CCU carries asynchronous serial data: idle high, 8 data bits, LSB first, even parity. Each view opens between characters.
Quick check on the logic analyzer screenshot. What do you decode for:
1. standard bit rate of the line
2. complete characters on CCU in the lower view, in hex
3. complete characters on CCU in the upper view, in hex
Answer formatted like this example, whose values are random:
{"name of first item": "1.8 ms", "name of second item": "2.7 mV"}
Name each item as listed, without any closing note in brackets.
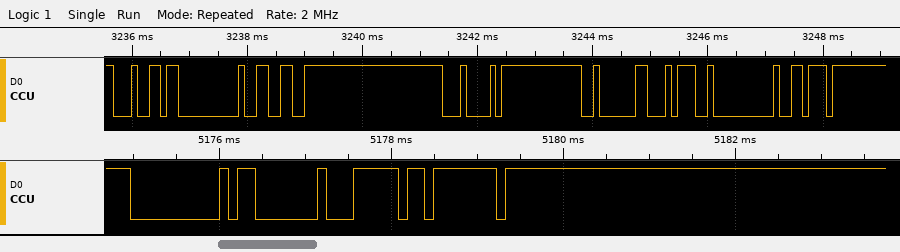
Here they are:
{"standard bit rate of the line": "9600 baud", "complete characters on CCU in the lower view, in hex": "00, 03, 7C, 7F", "complete characters on CCU in the upper view, in hex": "64, 00, 66, 84, 02, 74, 00, 76"}
